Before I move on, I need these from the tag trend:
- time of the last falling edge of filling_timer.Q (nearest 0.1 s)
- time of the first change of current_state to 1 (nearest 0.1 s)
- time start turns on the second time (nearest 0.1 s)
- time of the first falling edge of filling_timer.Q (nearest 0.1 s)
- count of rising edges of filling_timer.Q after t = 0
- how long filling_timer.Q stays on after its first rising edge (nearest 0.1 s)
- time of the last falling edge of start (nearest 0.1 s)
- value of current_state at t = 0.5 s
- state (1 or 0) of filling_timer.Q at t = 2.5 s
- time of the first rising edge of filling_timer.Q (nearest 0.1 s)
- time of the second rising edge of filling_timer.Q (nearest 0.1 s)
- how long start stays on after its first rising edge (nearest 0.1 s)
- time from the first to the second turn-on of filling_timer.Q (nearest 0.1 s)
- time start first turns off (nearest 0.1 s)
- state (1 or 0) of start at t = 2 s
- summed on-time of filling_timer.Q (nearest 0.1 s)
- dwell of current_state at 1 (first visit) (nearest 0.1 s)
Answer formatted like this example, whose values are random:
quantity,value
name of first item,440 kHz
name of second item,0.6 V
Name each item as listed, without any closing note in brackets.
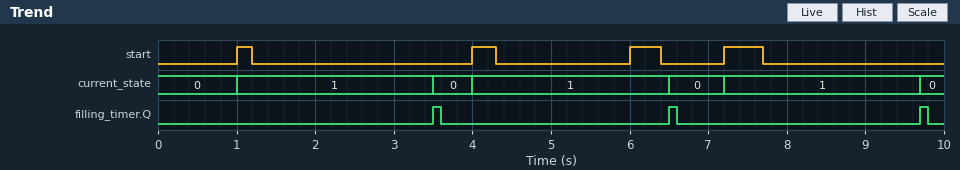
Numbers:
quantity,value
time of the last falling edge of filling_timer.Q,9.8 s
time of the first change of current_state to 1,1.0 s
time start turns on the second time,4.0 s
time of the first falling edge of filling_timer.Q,3.6 s
count of rising edges of filling_timer.Q after t = 0,3
how long filling_timer.Q stays on after its first rising edge,0.1 s
time of the last falling edge of start,7.7 s
value of current_state at t = 0.5 s,0
state (1 or 0) of filling_timer.Q at t = 2.5 s,0
time of the first rising edge of filling_timer.Q,3.5 s
time of the second rising edge of filling_timer.Q,6.5 s
how long start stays on after its first rising edge,0.2 s
time from the first to the second turn-on of filling_timer.Q,3.0 s
time start first turns off,1.2 s
state (1 or 0) of start at t = 2 s,0
summed on-time of filling_timer.Q,0.3 s
dwell of current_state at 1 (first visit),2.5 s
